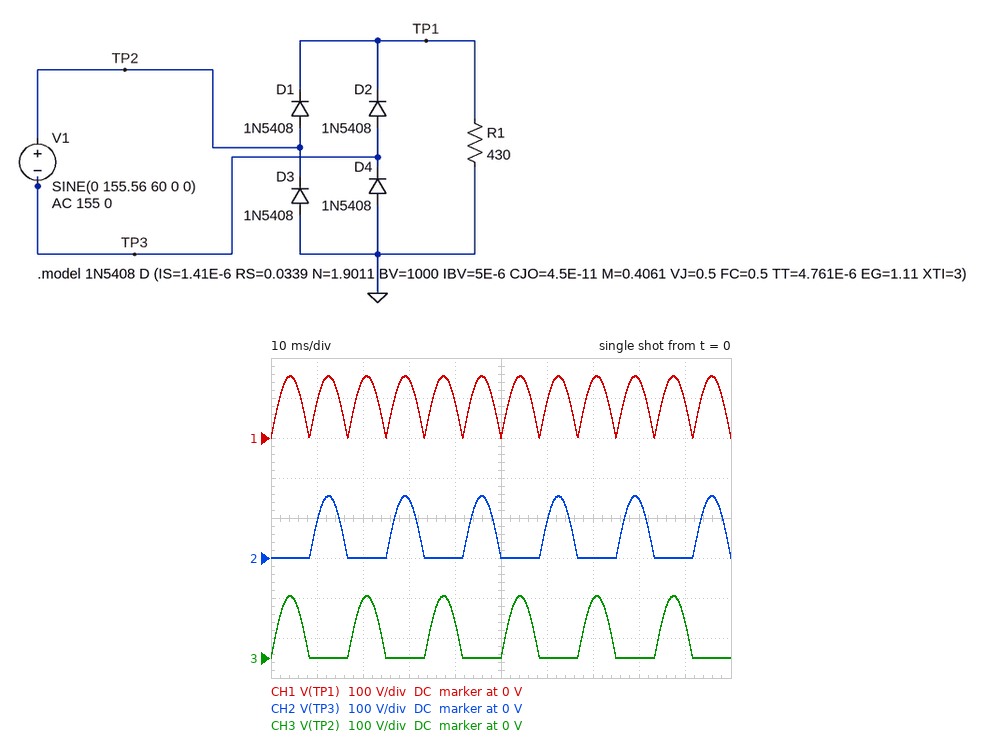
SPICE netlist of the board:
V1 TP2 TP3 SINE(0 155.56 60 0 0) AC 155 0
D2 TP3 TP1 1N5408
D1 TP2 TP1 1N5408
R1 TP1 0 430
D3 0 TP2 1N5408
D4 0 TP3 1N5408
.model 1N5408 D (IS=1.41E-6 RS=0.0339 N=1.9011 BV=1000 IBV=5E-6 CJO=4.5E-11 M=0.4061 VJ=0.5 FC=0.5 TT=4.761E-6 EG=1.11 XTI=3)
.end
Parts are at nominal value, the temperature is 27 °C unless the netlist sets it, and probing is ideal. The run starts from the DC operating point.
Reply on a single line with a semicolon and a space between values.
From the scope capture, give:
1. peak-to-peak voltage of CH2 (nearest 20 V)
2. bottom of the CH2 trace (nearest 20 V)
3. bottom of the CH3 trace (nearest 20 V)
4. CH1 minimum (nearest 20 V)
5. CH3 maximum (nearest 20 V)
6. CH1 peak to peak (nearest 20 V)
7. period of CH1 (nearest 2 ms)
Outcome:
160 V; 0 V; 0 V; 0 V; 160 V; 160 V; 8 ms
